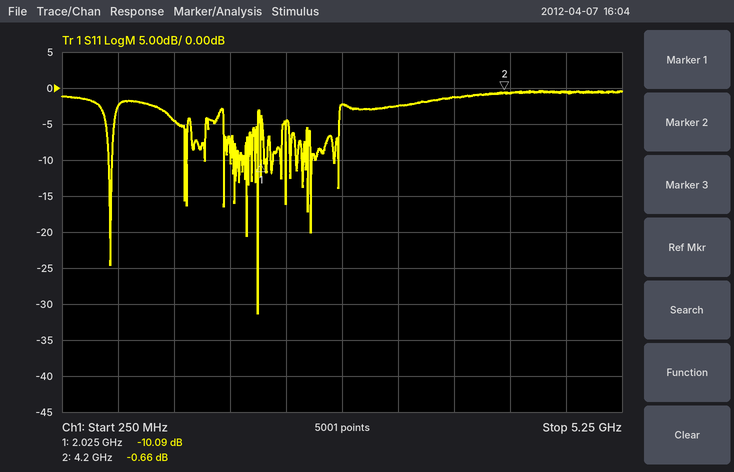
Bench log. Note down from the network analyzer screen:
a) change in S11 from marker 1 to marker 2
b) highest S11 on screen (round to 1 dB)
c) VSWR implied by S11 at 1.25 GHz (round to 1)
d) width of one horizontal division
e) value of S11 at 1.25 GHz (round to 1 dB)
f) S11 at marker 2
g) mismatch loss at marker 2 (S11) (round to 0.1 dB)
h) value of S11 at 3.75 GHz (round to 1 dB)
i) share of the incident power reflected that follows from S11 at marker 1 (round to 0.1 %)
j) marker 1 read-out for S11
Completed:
9.43 dB
0 dB
4
500 MHz
-5 dB
-0.66 dB
8.5 dB
-1 dB
9.8 %
-10.09 dB
